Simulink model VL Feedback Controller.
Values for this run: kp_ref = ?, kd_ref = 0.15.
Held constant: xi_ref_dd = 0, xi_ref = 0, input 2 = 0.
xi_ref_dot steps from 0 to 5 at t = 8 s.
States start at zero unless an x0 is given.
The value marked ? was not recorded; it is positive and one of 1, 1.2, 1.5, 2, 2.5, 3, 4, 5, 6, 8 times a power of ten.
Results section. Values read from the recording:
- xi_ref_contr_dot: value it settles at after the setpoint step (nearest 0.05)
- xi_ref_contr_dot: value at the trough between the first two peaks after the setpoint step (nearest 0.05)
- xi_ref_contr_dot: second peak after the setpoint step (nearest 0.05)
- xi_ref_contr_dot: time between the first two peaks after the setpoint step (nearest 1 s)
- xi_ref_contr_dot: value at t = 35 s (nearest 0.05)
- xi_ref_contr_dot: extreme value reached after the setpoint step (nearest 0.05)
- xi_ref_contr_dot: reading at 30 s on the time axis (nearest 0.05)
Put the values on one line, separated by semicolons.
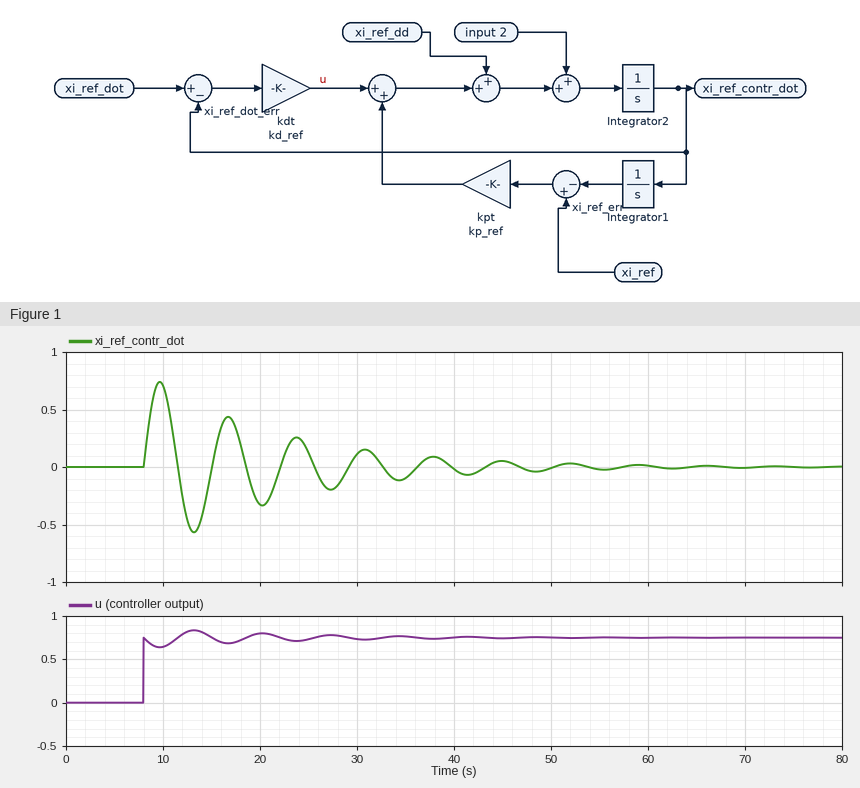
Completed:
0.00; -0.55; 0.45; 7 s; -0.10; 0.75; 0.10
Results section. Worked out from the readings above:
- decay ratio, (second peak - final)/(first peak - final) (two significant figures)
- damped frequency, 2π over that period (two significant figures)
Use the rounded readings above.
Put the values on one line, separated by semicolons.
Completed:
0.60; 0.90 rad/s
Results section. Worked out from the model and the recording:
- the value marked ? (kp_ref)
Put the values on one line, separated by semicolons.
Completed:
0.8
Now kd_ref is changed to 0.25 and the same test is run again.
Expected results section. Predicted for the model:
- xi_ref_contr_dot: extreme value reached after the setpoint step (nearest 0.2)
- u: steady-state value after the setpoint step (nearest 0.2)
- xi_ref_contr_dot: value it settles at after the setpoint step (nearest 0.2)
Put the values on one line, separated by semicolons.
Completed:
1.2; 1.2; 0.0
